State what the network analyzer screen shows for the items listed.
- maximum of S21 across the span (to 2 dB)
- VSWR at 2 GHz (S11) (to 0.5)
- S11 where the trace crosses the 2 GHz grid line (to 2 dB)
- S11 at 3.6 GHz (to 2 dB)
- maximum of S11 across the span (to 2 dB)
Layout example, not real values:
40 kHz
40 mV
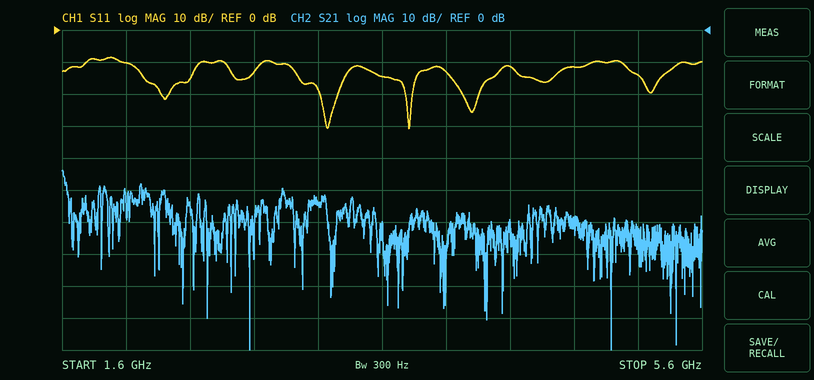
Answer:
-44 dB
2.0
-10 dB
-14 dB
-8 dB
